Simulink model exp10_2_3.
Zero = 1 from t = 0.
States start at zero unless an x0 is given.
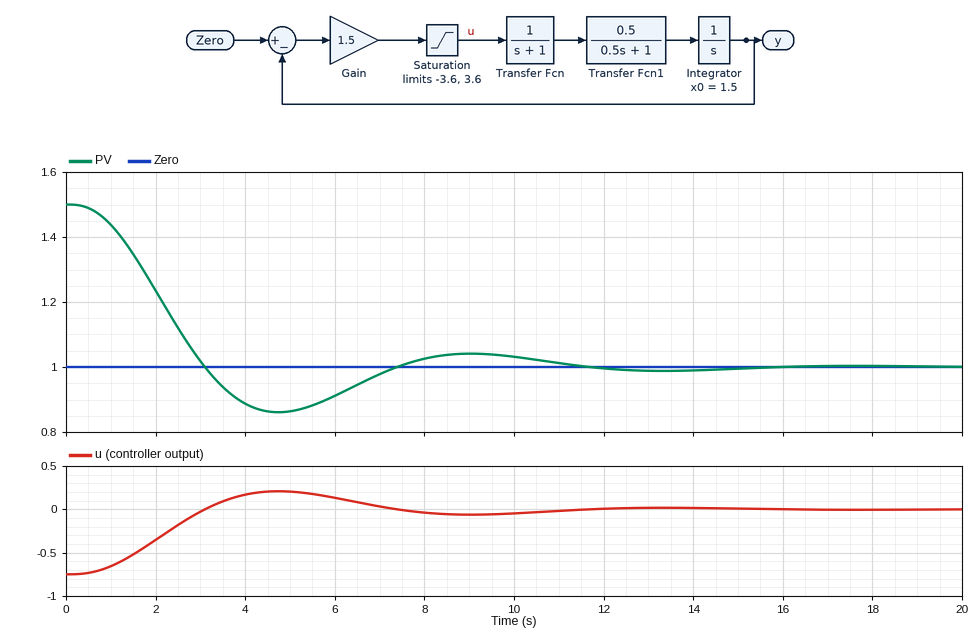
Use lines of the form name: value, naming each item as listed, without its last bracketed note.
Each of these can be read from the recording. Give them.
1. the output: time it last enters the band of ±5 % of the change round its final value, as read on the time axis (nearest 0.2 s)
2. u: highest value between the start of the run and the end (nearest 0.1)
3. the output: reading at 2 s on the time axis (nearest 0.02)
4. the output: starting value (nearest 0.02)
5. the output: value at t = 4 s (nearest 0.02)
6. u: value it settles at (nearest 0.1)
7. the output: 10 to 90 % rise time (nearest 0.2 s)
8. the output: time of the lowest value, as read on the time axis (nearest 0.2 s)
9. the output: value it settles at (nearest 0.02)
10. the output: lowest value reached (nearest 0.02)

the output: time it last enters the band of ±5 % of the change round its final value, as read on the time axis: 10.4 s
u: highest value between the start of the run and the end: 0.2
the output: reading at 2 s on the time axis: 1.24
the output: starting value: 1.50
the output: value at t = 4 s: 0.88
u: value it settles at: 0.0
the output: 10 to 90 % rise time: 2.0 s
the output: time of the lowest value, as read on the time axis: 4.8 s
the output: value it settles at: 1.00
the output: lowest value reached: 0.86
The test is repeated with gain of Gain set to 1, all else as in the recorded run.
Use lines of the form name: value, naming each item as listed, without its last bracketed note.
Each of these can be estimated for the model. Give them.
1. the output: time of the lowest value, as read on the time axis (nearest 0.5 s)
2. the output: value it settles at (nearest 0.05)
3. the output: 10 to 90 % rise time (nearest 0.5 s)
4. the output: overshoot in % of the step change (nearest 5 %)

the output: time of the lowest value, as read on the time axis: 6.0 s
the output: value it settles at: 1.00
the output: 10 to 90 % rise time: 2.5 s
the output: overshoot in % of the step change: 15 %
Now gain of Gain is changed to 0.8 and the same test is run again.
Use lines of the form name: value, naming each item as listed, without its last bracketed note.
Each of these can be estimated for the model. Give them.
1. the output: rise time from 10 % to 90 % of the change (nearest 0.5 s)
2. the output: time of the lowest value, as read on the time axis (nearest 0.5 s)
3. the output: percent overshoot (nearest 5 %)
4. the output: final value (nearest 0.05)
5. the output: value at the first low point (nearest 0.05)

the output: rise time from 10 % to 90 % of the change: 3.5 s
the output: time of the lowest value, as read on the time axis: 7.0 s
the output: percent overshoot: 10 %
the output: final value: 1.00
the output: value at the first low point: 0.95
